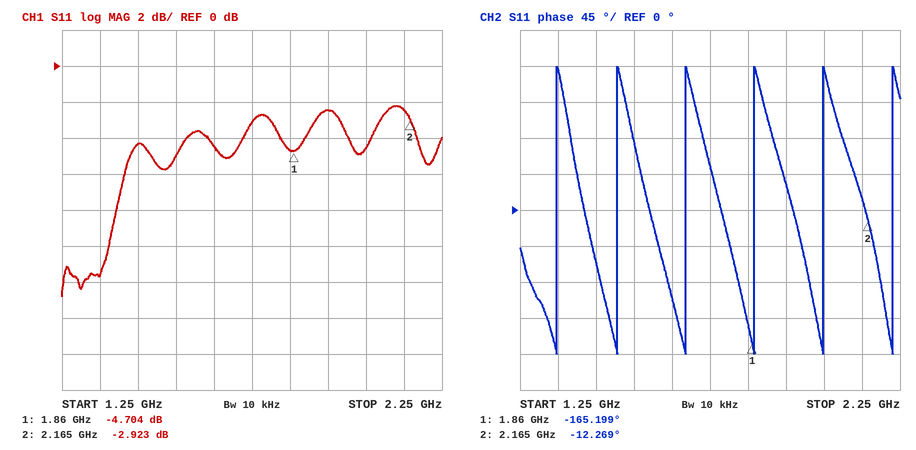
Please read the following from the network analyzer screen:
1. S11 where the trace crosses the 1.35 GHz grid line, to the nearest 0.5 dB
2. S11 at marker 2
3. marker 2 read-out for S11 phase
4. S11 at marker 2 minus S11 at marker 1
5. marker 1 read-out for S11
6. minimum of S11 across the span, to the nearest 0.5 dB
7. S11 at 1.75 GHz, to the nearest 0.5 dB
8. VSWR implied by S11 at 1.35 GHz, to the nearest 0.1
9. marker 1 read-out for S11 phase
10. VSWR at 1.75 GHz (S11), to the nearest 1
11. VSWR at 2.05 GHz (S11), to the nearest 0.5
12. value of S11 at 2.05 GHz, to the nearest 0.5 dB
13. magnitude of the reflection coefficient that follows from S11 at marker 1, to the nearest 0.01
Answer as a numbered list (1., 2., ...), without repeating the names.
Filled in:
1. -11.5 dB
2. -2.923 dB
3. -12.269°
4. 1.781 dB
5. -4.704 dB
6. -13.0 dB
7. -3.0 dB
8. 1.7
9. -165.199°
10. 6
11. 4.0
12. -4.5 dB
13. 0.58
